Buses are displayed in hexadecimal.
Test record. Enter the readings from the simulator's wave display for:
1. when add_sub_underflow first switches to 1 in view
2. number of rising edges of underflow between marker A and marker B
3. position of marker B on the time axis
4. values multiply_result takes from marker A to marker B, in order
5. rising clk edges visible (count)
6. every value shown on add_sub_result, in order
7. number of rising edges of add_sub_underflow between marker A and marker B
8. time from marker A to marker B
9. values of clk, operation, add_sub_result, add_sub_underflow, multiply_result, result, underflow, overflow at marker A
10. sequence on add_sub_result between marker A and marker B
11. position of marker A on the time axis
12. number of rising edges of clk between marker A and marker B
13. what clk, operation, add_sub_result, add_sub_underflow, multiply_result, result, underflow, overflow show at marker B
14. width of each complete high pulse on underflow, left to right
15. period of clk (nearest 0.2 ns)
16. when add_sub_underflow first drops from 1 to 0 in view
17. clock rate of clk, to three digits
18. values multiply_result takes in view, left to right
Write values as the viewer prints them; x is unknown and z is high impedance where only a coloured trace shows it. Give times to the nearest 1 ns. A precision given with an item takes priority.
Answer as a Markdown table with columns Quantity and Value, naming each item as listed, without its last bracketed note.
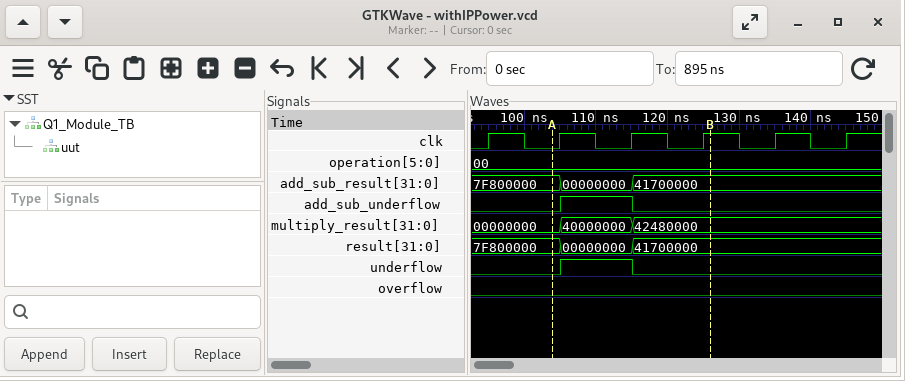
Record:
| Quantity | Value |
|---|---|
| when add_sub_underflow first switches to 1 in view | 105 ns |
| number of rising edges of underflow between marker A and marker B | 1 |
| position of marker B on the time axis | 126 ns |
| values multiply_result takes from marker A to marker B, in order | 00000000, 40000000, 42480000 |
| rising clk edges visible | 6 |
| every value shown on add_sub_result, in order | 7F800000, 00000000, 41700000 |
| number of rising edges of add_sub_underflow between marker A and marker B | 1 |
| time from marker A to marker B | 22 ns |
| values of clk, operation, add_sub_result, add_sub_underflow, multiply_result, result, underflow, overflow at marker A | clk=0, operation=00, add_sub_result=7F800000, add_sub_underflow=0, multiply_result=00000000, result=7F800000, underflow=0, overflow=0 |
| sequence on add_sub_result between marker A and marker B | 7F800000, 00000000, 41700000 |
| position of marker A on the time axis | 104 ns |
| number of rising edges of clk between marker A and marker B | 3 |
| what clk, operation, add_sub_result, add_sub_underflow, multiply_result, result, underflow, overflow show at marker B | clk=1, operation=00, add_sub_result=41700000, add_sub_underflow=0, multiply_result=42480000, result=41700000, underflow=0, overflow=0 |
| width of each complete high pulse on underflow, left to right | 10 ns |
| period of clk | 10 ns |
| when add_sub_underflow first drops from 1 to 0 in view | 115 ns |
| clock rate of clk, to three digits | 100 MHz |
| values multiply_result takes in view, left to right | 00000000, 40000000, 42480000 |
